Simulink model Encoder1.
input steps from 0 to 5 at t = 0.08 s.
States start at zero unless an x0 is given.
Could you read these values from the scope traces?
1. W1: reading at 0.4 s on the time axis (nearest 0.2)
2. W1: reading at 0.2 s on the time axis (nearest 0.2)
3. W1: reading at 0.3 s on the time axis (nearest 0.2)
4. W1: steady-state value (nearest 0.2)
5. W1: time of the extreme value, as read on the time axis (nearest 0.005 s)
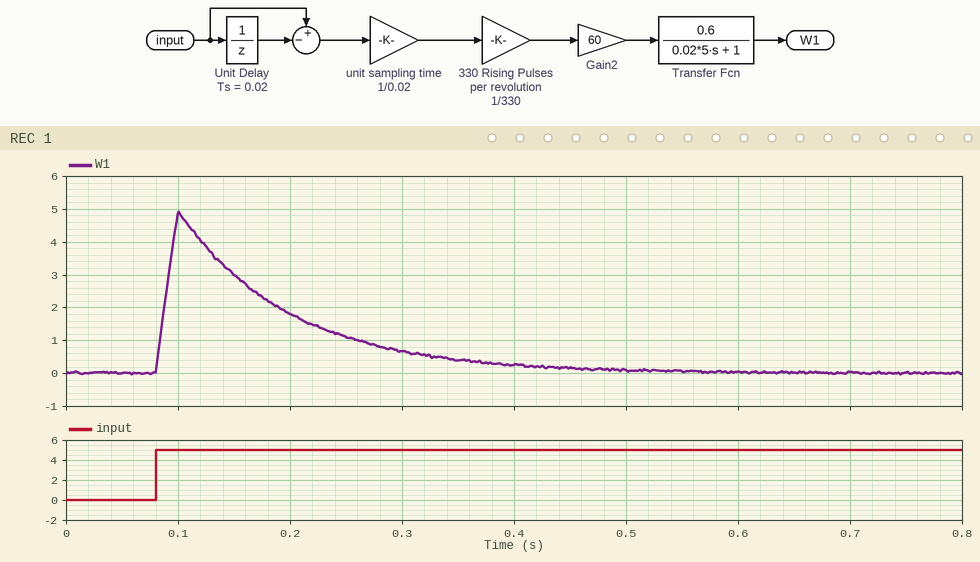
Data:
0.2
1.8
0.6
0.0
0.100 s
